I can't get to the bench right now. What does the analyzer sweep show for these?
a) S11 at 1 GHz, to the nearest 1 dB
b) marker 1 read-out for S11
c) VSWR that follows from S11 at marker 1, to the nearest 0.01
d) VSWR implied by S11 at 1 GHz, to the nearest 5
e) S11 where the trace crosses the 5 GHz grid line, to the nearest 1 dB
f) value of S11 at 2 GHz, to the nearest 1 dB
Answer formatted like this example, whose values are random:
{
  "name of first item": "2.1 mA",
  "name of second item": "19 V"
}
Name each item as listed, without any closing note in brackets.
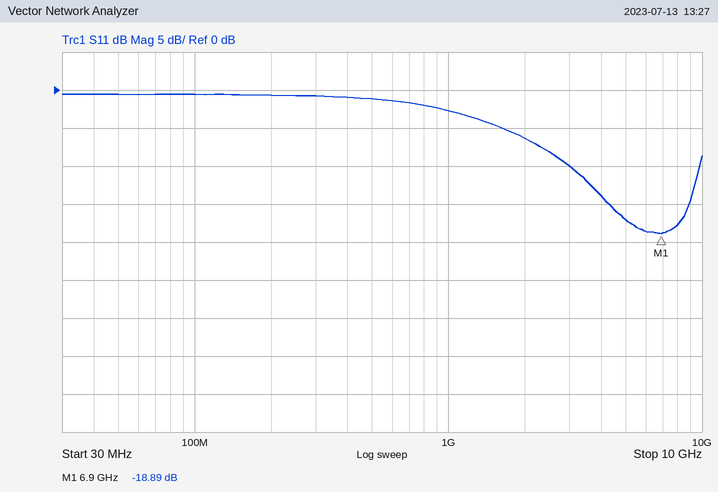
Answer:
{
  "S11 at 1 GHz, to the nearest 1 dB": "-3 dB",
  "marker 1 read-out for S11": "-18.89 dB",
  "VSWR that follows from S11 at marker 1, to the nearest 0.01": "1.26",
  "VSWR implied by S11 at 1 GHz, to the nearest 5": "5",
  "S11 where the trace crosses the 5 GHz grid line, to the nearest 1 dB": "-17 dB",
  "value of S11 at 2 GHz, to the nearest 1 dB": "-6 dB"
}
